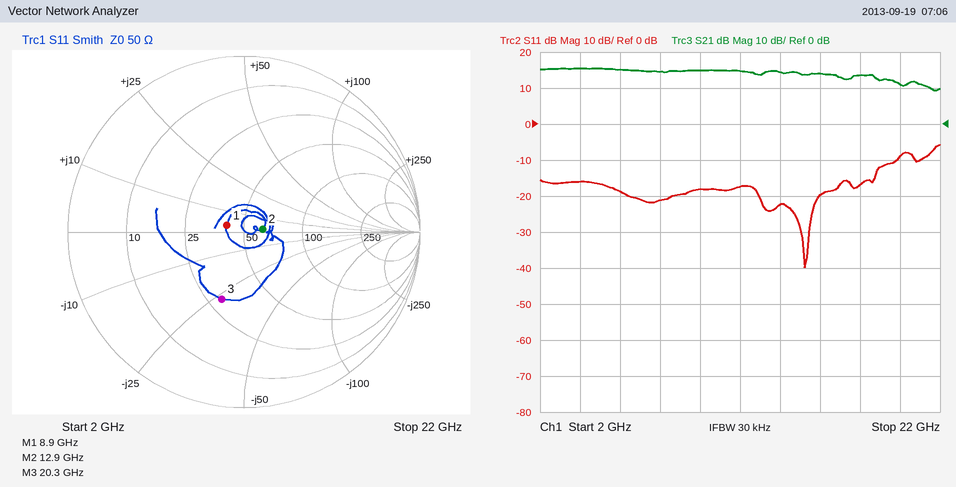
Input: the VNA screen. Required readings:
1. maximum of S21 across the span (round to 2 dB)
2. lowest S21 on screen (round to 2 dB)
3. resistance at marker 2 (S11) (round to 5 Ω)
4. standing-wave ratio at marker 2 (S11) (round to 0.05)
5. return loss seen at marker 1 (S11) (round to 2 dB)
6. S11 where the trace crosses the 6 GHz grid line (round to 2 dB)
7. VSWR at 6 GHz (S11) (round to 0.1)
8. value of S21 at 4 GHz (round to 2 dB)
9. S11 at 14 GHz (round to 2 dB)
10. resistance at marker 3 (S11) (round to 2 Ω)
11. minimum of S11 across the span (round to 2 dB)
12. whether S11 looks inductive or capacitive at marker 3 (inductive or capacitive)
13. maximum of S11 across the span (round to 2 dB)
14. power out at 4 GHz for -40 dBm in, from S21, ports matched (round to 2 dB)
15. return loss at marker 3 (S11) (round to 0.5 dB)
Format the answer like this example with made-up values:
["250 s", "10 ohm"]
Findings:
["16 dB", "10 dB", "60 Ω", "1.25", "20 dB", "-18 dB", "1.3", "16 dB", "-22 dB", "30 Ω", "-40 dB", "capacitive", "-6 dB", "-24 dBm", "8.0 dB"]
